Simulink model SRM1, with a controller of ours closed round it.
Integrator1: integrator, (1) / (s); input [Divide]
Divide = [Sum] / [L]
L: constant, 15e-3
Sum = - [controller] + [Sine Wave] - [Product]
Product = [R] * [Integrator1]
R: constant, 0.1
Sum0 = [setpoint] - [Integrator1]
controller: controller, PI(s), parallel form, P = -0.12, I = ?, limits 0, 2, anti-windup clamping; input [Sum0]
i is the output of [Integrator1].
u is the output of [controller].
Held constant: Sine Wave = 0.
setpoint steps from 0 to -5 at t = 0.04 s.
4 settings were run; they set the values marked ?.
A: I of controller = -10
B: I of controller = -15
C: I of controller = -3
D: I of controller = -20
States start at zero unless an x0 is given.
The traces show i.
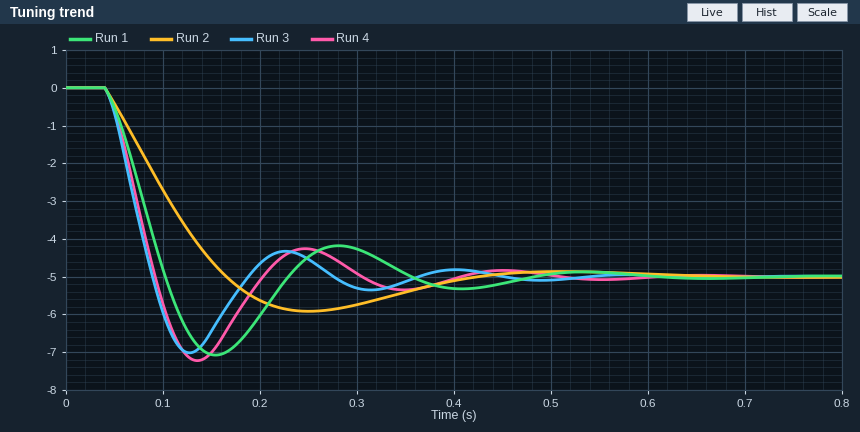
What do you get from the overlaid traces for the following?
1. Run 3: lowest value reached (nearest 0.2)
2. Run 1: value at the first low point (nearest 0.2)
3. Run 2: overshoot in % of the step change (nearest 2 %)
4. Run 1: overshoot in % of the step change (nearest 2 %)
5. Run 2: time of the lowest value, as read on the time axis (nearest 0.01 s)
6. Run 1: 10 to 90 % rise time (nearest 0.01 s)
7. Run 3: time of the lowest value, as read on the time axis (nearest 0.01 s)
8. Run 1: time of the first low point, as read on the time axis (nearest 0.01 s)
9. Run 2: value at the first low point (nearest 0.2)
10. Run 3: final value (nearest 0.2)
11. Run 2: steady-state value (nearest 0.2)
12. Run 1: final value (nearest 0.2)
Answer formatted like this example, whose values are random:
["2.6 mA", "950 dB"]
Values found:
["-7.0", "-7.0", "18 %", "42 %", "0.25 s", "0.05 s", "0.13 s", "0.15 s", "-6.0", "-5.0", "-5.0", "-5.0"]
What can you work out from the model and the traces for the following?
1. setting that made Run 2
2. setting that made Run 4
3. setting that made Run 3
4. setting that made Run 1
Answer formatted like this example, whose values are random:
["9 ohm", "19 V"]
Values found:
["C", "B", "D", "A"]
